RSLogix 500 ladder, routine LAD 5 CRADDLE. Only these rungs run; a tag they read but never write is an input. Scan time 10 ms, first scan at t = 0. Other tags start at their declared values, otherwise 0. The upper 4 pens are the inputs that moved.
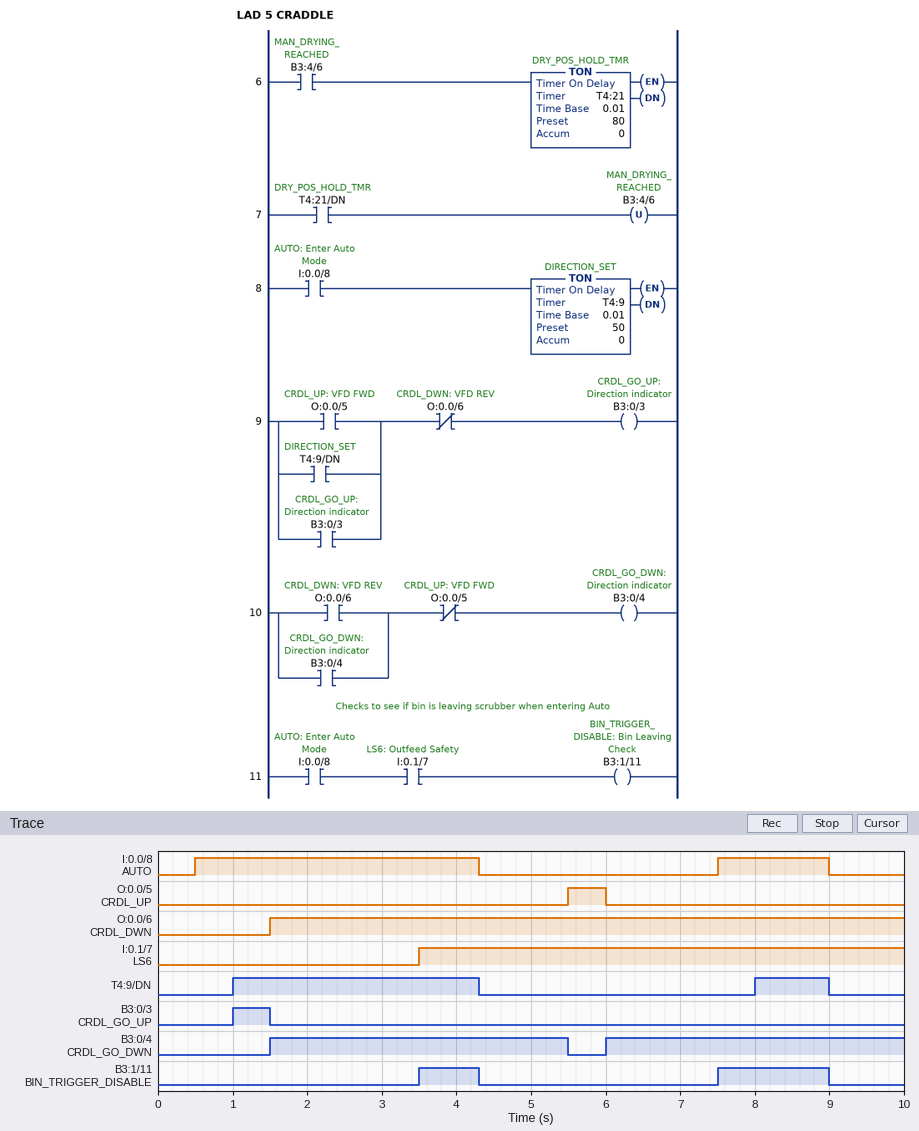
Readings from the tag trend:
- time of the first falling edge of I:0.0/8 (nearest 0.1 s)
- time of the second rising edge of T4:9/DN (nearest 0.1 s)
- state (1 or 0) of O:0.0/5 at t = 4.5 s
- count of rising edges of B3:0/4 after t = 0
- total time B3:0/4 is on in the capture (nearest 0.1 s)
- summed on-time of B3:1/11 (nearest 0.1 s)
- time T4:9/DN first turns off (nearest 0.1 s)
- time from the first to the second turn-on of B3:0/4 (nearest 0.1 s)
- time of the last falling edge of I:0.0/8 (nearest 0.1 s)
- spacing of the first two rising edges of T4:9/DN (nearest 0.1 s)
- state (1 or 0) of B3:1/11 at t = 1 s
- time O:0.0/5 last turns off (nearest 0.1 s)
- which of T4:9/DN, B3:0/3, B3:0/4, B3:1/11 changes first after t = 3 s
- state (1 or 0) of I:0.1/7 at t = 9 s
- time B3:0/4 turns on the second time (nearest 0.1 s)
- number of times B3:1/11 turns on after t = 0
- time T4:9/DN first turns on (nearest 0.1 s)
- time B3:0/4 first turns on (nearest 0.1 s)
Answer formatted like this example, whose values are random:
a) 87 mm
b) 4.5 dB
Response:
a) 4.3 s
b) 8.0 s
c) 0
d) 2
e) 8.0 s
f) 2.3 s
g) 4.3 s
h) 4.5 s
i) 9.0 s
j) 7.0 s
k) 0
l) 6.0 s
m) B3:1/11
n) 1
o) 6.0 s
p) 2
q) 1.0 s
r) 1.5 s
